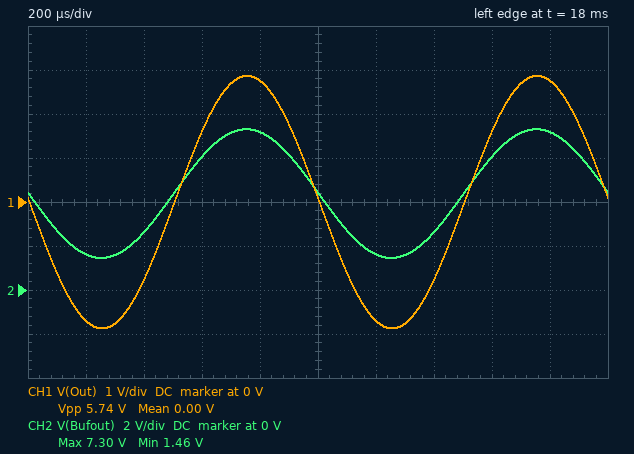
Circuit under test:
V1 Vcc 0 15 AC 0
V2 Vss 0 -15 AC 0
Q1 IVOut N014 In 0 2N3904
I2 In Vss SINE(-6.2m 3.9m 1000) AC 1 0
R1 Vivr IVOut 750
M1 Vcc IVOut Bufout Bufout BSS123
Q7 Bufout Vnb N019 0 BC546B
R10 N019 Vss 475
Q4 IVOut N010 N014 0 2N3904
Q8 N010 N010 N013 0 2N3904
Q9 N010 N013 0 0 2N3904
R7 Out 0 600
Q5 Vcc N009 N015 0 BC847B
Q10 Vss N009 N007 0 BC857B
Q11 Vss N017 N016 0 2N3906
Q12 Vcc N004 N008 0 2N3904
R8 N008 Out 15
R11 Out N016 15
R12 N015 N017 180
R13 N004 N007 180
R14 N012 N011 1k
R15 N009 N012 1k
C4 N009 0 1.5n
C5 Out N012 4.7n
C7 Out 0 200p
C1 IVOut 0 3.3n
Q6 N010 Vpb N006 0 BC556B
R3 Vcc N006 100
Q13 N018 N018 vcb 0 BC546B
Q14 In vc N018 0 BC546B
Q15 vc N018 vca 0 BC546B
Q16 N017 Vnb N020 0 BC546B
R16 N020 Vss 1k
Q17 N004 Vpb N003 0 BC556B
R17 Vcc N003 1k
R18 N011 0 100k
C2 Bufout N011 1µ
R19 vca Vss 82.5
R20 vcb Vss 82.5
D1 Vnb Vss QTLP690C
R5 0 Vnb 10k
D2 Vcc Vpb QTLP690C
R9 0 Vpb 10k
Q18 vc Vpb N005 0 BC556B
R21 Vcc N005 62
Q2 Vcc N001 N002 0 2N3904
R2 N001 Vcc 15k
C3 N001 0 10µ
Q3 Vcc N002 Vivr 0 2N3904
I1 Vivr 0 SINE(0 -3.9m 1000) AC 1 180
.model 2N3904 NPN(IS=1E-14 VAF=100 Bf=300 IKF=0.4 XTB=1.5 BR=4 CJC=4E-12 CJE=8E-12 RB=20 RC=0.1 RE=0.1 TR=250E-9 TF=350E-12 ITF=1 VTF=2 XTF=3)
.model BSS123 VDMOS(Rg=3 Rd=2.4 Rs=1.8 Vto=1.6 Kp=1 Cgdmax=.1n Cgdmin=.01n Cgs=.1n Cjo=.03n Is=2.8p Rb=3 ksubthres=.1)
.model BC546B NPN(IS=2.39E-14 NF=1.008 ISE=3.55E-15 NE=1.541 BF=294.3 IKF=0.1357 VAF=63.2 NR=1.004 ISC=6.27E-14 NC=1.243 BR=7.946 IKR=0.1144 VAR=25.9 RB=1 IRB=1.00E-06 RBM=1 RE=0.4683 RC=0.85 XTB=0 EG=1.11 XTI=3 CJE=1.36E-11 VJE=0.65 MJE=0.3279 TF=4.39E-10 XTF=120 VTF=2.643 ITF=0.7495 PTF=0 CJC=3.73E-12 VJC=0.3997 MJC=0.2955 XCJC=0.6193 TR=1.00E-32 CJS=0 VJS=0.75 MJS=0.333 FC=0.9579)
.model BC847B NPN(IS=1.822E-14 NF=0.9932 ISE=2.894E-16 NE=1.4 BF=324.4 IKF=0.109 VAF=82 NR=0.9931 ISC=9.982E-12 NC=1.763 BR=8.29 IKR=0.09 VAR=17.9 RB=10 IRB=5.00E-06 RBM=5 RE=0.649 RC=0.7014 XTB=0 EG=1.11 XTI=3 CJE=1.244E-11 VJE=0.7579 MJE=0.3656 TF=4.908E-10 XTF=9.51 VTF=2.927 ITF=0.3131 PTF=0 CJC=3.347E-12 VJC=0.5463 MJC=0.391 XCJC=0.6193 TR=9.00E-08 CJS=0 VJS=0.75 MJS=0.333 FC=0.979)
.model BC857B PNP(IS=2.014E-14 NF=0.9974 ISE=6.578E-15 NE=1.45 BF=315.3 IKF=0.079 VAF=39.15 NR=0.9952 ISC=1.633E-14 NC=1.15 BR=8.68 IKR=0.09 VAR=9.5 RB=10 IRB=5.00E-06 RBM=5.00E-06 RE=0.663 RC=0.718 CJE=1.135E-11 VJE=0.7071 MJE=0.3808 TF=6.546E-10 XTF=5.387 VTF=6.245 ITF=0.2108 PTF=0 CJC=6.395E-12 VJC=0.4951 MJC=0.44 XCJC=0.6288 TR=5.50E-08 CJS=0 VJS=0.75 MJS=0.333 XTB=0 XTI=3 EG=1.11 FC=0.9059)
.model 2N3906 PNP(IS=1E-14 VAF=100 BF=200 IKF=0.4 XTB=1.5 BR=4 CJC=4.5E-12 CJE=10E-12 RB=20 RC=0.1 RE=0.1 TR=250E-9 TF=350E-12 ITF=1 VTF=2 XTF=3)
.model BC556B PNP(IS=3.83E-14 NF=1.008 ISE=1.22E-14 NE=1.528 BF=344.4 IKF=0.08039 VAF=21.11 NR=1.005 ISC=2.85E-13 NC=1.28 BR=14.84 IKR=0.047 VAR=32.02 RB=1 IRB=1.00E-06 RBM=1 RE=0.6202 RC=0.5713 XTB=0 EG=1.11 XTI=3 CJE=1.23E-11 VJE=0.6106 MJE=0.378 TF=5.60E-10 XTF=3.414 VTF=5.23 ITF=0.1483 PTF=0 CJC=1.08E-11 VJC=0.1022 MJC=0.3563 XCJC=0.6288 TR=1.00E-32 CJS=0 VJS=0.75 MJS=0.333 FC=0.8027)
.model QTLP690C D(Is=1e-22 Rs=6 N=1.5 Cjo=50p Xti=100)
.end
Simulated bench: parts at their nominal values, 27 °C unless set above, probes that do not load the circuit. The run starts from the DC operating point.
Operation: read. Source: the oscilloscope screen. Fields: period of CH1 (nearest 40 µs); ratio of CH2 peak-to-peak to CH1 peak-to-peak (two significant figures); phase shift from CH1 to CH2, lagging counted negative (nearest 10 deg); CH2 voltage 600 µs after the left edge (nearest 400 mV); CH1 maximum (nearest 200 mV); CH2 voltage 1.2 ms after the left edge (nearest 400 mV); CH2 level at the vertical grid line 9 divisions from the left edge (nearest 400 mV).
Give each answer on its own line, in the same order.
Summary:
1.00 ms
1.0
0 deg
6.0 V
2.8 V
1.6 V
7.2 V
